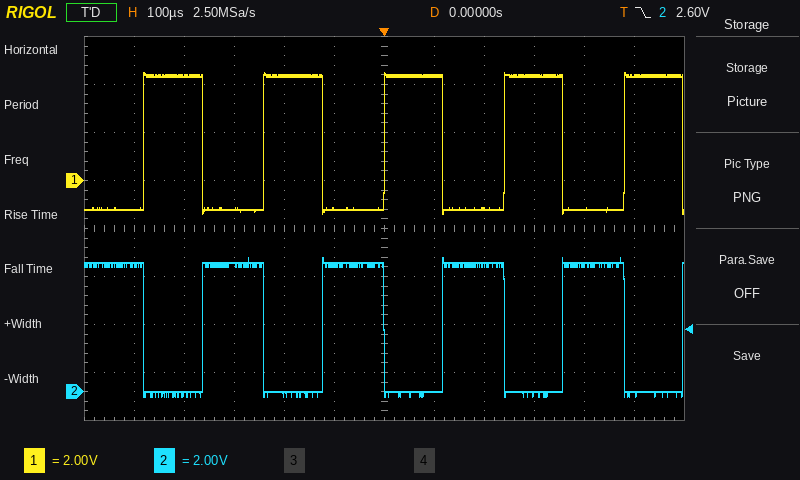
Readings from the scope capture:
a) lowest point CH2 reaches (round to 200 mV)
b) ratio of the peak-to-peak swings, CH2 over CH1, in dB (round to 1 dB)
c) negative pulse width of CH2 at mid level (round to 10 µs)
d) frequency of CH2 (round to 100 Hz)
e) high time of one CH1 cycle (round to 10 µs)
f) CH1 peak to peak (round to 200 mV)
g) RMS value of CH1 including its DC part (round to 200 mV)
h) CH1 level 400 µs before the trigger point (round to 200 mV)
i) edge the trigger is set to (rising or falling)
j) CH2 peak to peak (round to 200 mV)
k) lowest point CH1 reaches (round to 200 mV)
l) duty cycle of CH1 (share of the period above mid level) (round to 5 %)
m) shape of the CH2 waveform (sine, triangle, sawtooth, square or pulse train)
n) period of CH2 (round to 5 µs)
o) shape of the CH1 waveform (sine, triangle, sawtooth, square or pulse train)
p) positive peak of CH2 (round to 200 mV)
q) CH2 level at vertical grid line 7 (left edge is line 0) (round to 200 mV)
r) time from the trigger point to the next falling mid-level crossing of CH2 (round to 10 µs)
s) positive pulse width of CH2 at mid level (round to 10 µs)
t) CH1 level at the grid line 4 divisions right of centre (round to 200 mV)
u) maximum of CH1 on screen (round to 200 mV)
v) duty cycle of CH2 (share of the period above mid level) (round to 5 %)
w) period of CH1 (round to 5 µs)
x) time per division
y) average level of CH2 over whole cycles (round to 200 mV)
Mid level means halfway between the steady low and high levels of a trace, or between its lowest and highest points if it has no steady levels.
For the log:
-200 mV
0 dB
120 µs
4.2 kHz
120 µs
5.8 V
3.2 V
4.4 V
falling
5.8 V
-1.4 V
50 %
square
240 µs
square
5.6 V
0.0 V
240 µs
120 µs
-1.2 V
4.4 V
50 %
240 µs
100 µs
2.8 V
